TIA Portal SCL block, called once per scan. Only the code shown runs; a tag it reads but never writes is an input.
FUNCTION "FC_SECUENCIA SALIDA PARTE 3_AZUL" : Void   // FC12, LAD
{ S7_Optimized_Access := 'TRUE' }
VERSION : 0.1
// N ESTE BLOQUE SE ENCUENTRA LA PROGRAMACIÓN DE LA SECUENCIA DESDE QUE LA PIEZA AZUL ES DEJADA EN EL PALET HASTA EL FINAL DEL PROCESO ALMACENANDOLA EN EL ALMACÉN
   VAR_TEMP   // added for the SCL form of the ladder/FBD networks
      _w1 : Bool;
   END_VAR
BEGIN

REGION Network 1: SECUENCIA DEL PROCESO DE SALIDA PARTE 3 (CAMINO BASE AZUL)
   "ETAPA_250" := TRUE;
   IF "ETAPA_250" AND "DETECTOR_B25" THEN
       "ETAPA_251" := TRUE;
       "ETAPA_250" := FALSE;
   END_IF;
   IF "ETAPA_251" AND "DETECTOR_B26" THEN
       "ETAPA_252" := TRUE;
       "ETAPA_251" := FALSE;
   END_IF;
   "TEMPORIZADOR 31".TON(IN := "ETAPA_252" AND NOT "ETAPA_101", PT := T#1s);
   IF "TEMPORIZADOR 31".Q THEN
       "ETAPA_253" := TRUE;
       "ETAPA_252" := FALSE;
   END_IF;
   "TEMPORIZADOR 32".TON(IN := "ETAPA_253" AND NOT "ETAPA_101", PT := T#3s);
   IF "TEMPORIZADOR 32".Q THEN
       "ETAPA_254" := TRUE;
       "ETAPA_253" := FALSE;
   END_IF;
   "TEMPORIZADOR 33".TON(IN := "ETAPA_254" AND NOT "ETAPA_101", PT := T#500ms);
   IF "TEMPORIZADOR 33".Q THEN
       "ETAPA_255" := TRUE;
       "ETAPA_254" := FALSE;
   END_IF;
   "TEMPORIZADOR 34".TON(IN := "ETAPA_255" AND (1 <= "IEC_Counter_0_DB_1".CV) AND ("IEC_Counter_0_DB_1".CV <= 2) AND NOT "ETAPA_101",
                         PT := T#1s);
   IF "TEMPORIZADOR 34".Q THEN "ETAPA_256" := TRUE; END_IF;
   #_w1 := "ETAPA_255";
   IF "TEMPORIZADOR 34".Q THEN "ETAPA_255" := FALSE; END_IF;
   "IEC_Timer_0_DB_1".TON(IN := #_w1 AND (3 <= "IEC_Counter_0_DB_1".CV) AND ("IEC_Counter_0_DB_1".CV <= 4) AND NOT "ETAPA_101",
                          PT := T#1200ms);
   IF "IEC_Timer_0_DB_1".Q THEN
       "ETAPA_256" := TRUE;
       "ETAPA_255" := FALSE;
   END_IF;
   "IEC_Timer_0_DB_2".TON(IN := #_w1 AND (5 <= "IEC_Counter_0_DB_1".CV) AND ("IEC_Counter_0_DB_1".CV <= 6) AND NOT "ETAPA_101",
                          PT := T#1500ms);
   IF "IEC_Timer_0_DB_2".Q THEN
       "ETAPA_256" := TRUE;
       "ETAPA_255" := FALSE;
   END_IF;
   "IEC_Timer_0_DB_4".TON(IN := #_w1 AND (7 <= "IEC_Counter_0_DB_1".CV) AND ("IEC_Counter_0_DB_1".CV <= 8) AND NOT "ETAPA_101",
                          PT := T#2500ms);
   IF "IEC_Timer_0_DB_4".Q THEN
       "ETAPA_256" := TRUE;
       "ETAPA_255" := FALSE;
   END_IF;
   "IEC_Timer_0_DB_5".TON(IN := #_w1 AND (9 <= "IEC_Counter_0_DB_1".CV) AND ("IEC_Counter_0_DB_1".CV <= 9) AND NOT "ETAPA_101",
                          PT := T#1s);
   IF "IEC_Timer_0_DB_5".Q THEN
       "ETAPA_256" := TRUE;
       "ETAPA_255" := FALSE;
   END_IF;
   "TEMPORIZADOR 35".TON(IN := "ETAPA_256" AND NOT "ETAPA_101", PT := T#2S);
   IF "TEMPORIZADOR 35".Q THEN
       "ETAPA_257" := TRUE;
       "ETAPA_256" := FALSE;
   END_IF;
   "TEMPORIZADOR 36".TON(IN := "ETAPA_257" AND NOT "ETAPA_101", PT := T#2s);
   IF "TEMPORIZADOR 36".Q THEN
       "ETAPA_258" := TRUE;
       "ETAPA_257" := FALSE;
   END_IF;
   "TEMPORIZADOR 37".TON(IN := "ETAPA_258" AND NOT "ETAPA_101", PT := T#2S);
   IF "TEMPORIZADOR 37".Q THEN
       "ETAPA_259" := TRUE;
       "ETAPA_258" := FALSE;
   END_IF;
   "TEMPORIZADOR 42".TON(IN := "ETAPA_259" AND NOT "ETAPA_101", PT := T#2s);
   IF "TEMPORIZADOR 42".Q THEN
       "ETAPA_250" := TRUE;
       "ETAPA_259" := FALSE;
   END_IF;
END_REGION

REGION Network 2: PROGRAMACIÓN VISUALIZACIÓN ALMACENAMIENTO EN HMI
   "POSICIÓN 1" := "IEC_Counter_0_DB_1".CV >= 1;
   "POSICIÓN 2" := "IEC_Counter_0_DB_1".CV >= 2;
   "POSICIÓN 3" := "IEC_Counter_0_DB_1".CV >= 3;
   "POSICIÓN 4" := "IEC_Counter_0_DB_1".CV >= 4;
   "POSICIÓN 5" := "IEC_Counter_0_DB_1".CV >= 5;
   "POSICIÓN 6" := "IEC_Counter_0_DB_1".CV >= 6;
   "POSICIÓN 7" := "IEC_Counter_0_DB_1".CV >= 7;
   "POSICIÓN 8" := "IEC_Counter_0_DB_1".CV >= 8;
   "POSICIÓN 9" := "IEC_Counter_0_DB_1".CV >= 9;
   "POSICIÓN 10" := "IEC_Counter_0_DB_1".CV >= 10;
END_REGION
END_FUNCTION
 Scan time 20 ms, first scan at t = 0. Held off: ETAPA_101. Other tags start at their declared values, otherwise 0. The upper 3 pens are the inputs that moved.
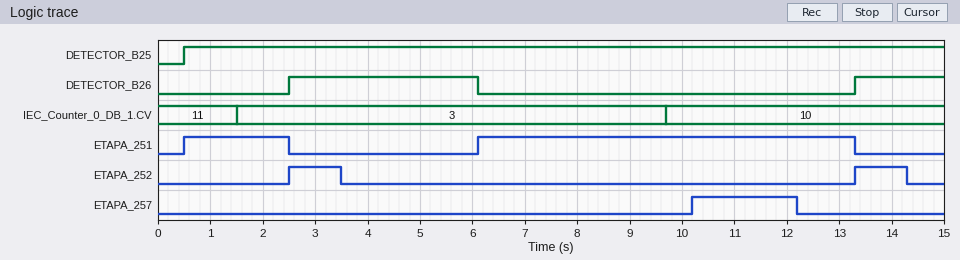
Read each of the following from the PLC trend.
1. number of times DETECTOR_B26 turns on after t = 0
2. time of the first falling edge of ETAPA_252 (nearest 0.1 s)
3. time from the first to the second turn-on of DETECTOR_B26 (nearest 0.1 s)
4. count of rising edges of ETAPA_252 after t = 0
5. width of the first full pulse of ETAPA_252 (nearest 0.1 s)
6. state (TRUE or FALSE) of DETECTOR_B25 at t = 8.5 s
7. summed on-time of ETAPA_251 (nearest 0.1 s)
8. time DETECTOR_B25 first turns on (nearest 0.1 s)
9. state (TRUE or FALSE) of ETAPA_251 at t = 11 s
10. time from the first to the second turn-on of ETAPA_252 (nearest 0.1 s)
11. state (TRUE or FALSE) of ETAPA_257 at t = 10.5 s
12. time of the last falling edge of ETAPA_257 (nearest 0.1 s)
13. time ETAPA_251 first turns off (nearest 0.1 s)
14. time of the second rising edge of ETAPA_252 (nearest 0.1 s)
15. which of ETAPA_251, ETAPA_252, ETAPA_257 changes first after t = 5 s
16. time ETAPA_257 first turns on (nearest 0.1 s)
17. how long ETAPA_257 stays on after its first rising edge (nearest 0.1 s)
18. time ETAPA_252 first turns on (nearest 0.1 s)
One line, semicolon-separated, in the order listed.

2; 3.5 s; 10.8 s; 2; 1.0 s; TRUE; 9.2 s; 0.5 s; TRUE; 10.8 s; TRUE; 12.2 s; 2.5 s; 13.3 s; ETAPA_251; 10.2 s; 2.0 s; 2.5 s
